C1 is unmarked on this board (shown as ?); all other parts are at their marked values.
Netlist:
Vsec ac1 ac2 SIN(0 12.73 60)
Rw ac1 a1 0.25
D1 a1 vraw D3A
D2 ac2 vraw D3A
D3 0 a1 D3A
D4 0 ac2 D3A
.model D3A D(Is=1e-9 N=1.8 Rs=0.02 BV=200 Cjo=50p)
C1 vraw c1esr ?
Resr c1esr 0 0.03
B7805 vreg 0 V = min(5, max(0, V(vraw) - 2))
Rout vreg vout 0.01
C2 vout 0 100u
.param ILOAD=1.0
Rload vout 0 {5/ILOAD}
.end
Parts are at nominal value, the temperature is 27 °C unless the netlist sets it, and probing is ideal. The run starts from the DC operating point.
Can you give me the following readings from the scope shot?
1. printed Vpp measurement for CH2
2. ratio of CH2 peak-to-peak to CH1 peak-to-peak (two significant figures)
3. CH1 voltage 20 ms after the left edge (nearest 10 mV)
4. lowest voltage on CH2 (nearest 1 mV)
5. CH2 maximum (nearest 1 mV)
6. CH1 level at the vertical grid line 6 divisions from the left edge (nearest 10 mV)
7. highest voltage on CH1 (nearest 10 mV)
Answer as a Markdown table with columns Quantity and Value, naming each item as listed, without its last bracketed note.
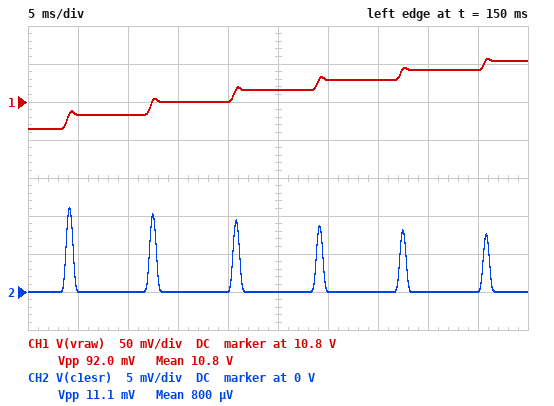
| Quantity | Value |
|---|---|
| printed Vpp measurement for CH2 | 11.1 mV |
| ratio of CH2 peak-to-peak to CH1 peak-to-peak | 0.12 |
| CH1 voltage 20 ms after the left edge | 10.80 V |
| lowest voltage on CH2 | 0 V |
| CH2 maximum | 11 mV |
| CH1 level at the vertical grid line 6 divisions from the left edge | 10.83 V |
| highest voltage on CH1 | 10.86 V |
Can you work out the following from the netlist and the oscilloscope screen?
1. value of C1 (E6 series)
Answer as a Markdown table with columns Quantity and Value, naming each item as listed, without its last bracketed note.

| Quantity | Value |
|---|---|
| value of C1 | 15 mF |
